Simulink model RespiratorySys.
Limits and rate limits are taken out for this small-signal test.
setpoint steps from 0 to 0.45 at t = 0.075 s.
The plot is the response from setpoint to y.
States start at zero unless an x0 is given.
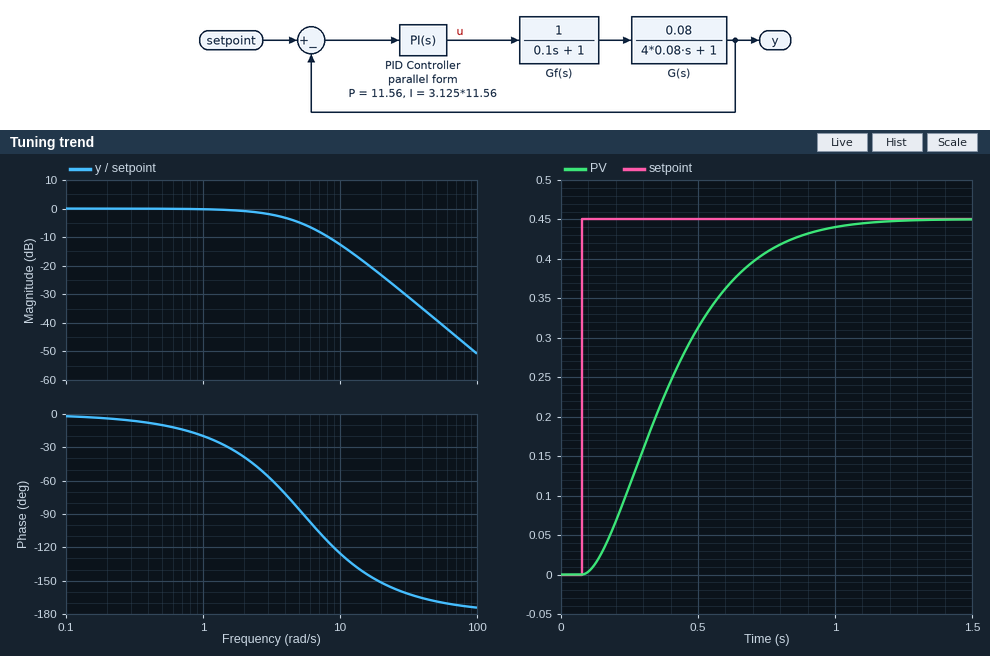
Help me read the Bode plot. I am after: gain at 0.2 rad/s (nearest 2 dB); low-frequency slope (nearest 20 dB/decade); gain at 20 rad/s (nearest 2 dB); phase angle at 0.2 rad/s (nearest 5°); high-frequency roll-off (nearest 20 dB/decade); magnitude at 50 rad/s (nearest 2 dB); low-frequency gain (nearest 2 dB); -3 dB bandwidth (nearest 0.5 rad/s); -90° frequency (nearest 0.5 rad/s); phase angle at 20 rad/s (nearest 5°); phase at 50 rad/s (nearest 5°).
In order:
0 dB
0 dB/decade
-24 dB
-5°
-40 dB/decade
-38 dB
0 dB
4.0 rad/s
5.5 rad/s
-150°
-170°
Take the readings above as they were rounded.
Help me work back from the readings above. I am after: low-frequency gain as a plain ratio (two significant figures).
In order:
1.0
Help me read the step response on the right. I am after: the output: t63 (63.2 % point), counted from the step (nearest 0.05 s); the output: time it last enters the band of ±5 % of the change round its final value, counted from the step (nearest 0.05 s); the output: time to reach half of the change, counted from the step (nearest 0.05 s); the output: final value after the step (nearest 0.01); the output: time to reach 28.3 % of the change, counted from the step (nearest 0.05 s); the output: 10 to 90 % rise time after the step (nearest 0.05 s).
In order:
0.40 s
0.80 s
0.30 s
0.45
0.20 s
0.55 s
